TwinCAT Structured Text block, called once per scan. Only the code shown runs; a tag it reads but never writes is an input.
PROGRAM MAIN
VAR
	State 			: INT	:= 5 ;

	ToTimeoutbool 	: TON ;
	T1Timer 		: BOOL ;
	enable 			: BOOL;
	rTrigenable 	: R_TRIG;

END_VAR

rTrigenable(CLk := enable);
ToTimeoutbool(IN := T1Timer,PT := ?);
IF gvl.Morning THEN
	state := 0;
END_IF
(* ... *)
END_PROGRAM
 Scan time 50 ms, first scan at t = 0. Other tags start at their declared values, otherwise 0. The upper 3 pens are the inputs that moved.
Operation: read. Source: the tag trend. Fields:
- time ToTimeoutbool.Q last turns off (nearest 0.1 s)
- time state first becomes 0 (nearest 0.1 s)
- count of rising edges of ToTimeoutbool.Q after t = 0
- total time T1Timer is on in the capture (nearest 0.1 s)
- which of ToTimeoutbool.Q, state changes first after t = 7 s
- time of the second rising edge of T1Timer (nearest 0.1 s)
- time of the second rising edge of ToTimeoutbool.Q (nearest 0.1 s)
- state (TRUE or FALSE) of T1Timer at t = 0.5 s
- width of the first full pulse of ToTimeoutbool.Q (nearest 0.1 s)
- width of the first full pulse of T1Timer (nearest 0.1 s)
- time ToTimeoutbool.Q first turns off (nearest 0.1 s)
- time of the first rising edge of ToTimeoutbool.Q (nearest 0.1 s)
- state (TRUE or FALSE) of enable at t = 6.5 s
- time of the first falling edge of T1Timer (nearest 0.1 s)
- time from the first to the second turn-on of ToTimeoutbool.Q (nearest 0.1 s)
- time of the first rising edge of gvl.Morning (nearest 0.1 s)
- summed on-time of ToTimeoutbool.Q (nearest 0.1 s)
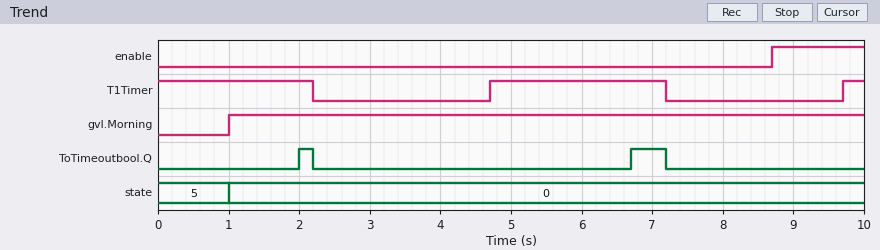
7.2 s
1.0 s
2
5.0 s
ToTimeoutbool.Q
9.7 s
6.7 s
TRUE
0.2 s
2.5 s
2.2 s
2.0 s
FALSE
2.2 s
4.7 s
1.0 s
0.7 s
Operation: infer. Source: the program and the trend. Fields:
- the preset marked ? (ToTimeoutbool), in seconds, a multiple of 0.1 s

2.0 s
